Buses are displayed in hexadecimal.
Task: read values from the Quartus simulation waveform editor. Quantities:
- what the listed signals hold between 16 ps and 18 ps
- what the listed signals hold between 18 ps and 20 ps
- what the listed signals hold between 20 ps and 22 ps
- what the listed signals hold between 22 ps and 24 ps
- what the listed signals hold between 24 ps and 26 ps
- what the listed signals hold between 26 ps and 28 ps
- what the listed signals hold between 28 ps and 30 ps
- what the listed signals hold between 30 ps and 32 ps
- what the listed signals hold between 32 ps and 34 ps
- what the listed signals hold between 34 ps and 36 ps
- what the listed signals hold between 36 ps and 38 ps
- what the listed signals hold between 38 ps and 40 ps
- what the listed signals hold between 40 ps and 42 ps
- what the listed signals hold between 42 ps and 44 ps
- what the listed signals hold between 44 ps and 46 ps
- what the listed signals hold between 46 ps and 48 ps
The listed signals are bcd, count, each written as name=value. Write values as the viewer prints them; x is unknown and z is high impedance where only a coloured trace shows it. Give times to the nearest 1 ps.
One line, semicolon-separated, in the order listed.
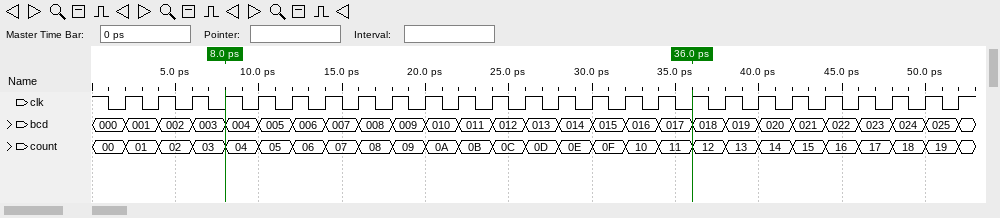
bcd=008, count=08; bcd=009, count=09; bcd=010, count=0A; bcd=011, count=0B; bcd=012, count=0C; bcd=013, count=0D; bcd=014, count=0E; bcd=015, count=0F; bcd=016, count=10; bcd=017, count=11; bcd=018, count=12; bcd=019, count=13; bcd=020, count=14; bcd=021, count=15; bcd=022, count=16; bcd=023, count=17
